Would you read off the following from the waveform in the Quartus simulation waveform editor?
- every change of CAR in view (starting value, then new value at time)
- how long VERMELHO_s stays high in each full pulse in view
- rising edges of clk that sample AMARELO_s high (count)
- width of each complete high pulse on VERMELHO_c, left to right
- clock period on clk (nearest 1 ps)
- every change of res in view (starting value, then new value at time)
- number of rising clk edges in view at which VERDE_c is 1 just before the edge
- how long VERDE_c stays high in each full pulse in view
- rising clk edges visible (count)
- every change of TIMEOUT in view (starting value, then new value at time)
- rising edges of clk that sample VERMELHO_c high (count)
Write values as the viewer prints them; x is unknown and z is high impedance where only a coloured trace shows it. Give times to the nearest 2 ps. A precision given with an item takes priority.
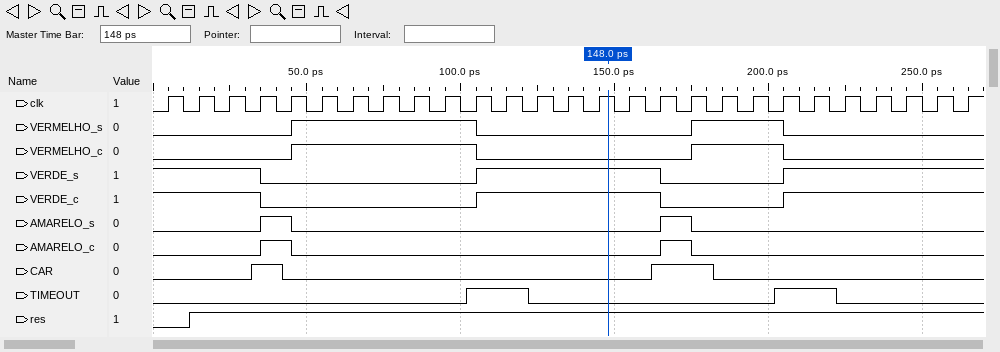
0, 1 at 32 ps, 0 at 42 ps, 1 at 162 ps, 0 at 182 ps
60 ps, 30 ps
2
60 ps, 30 ps
10 ps
0, 1 at 12 ps
16
60 ps
27
0, 1 at 102 ps, 0 at 122 ps, 1 at 202 ps, 0 at 222 ps
9
